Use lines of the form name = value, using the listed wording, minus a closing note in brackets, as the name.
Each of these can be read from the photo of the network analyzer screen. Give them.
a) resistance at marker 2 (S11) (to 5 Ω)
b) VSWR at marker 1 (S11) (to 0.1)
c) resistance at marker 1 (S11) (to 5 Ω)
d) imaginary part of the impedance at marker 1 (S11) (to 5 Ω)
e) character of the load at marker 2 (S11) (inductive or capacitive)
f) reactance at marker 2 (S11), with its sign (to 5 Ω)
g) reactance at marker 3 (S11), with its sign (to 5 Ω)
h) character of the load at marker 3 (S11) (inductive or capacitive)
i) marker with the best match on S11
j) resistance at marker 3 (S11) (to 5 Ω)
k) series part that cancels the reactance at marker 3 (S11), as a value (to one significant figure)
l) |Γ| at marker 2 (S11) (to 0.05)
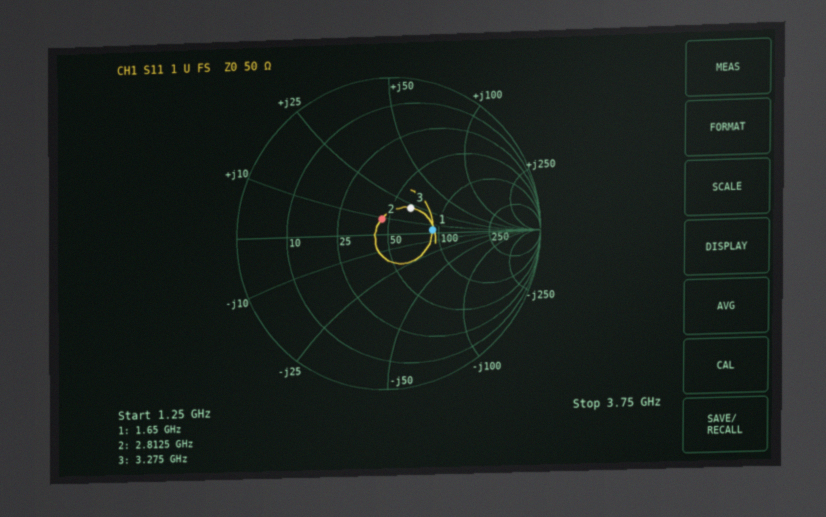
resistance at marker 2 (S11) = 45 Ω
VSWR at marker 1 (S11) = 1.8
resistance at marker 1 (S11) = 90 Ω
imaginary part of the impedance at marker 1 (S11) = +5 Ω
character of the load at marker 2 (S11) = inductive
reactance at marker 2 (S11), with its sign = +10 Ω
reactance at marker 3 (S11), with its sign = +20 Ω
character of the load at marker 3 (S11) = inductive
marker with the best match on S11 = marker 2
resistance at marker 3 (S11) = 65 Ω
series part that cancels the reactance at marker 3 (S11), as a value = 2 pF
|Γ| at marker 2 (S11) = 0.10
